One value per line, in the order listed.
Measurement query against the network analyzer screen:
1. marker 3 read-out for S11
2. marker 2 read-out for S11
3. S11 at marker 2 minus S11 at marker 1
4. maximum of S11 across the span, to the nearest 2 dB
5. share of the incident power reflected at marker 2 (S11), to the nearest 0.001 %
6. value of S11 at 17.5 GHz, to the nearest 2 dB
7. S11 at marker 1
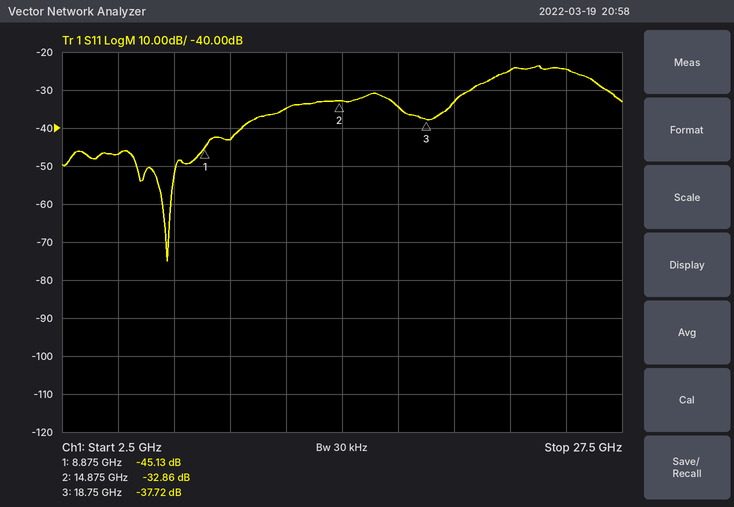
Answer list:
-37.72 dB
-32.86 dB
12.27 dB
-24 dB
0.052 %
-34 dB
-45.13 dB
